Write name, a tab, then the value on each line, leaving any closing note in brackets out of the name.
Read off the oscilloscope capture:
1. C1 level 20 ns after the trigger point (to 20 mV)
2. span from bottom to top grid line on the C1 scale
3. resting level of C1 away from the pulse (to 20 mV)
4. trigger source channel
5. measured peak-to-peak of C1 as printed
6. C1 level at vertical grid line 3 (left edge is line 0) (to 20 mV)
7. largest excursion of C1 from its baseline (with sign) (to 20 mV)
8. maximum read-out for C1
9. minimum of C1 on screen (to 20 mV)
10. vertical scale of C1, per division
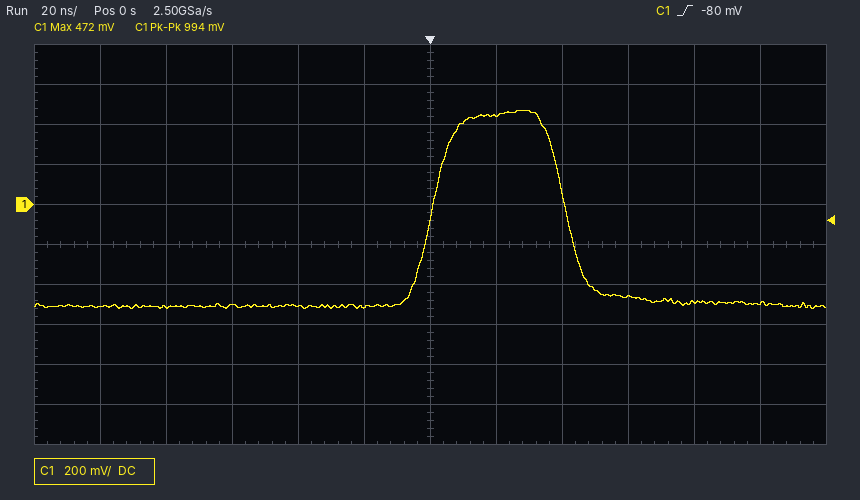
C1 level 20 ns after the trigger point	440 mV
span from bottom to top grid line on the C1 scale	2 V
resting level of C1 away from the pulse	-500 mV
trigger source channel	C1
measured peak-to-peak of C1 as printed	994 mV
C1 level at vertical grid line 3 (left edge is line 0)	-500 mV
largest excursion of C1 from its baseline (with sign)	+980 mV
maximum read-out for C1	472 mV
minimum of C1 on screen	-520 mV
vertical scale of C1, per division	200 mV
